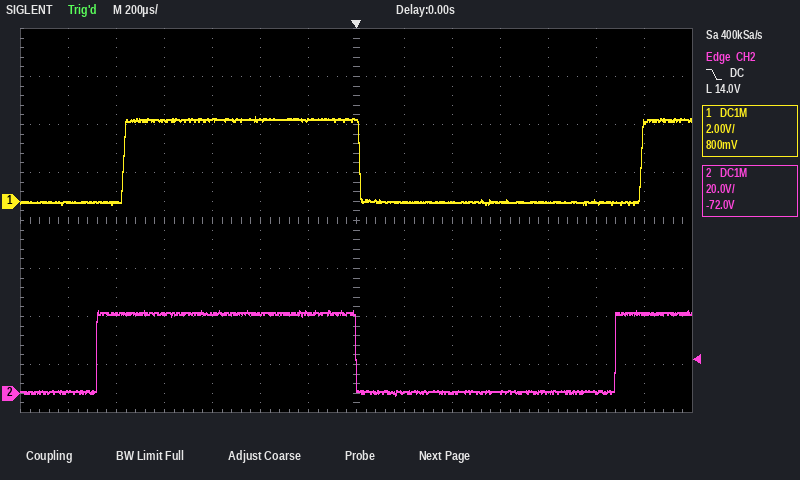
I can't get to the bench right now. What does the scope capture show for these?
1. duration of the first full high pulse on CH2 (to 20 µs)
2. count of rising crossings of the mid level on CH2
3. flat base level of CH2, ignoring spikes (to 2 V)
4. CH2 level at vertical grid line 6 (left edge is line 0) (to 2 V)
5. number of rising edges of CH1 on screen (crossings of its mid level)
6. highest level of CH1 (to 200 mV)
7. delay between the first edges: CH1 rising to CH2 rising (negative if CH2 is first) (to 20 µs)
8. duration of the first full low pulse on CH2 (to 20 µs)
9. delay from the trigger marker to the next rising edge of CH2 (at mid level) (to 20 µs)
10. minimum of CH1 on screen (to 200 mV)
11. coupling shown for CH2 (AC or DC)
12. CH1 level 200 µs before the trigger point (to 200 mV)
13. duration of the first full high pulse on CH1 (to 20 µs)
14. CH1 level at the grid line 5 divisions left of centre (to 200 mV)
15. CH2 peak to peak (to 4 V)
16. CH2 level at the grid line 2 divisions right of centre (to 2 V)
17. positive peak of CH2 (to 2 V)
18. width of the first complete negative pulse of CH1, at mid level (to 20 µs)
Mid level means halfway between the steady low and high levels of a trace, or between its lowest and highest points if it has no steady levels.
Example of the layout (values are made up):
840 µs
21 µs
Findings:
1.08 ms
2
0 V
34 V
2
3.6 V
-120 µs
1.08 ms
1.08 ms
-200 mV
DC
3.4 V
980 µs
0.0 V
36 V
0 V
34 V
1.18 ms
